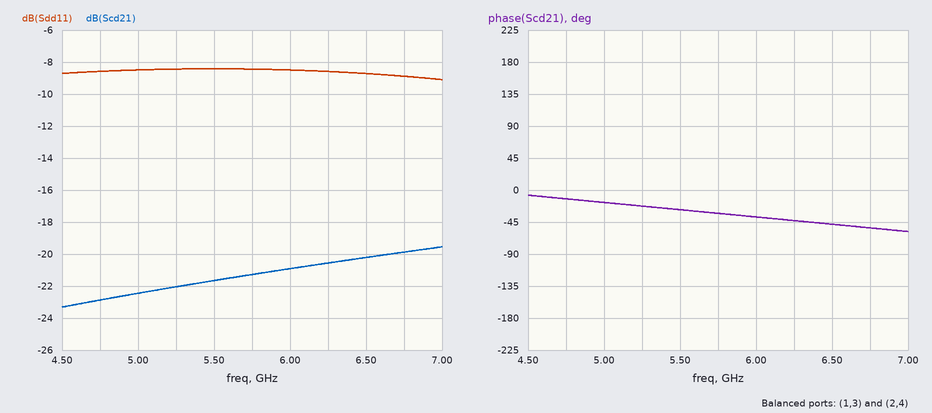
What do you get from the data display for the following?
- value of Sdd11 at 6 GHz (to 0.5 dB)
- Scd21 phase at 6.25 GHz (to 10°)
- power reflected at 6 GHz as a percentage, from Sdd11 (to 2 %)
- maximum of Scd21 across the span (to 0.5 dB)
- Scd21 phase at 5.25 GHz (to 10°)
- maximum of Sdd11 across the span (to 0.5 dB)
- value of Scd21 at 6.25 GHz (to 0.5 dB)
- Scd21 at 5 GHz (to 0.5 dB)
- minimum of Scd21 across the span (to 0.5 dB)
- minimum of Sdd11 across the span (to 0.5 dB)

-8.5 dB
-40°
14 %
-19.5 dB
-20°
-8.5 dB
-20.5 dB
-22.5 dB
-23.5 dB
-9.0 dB
